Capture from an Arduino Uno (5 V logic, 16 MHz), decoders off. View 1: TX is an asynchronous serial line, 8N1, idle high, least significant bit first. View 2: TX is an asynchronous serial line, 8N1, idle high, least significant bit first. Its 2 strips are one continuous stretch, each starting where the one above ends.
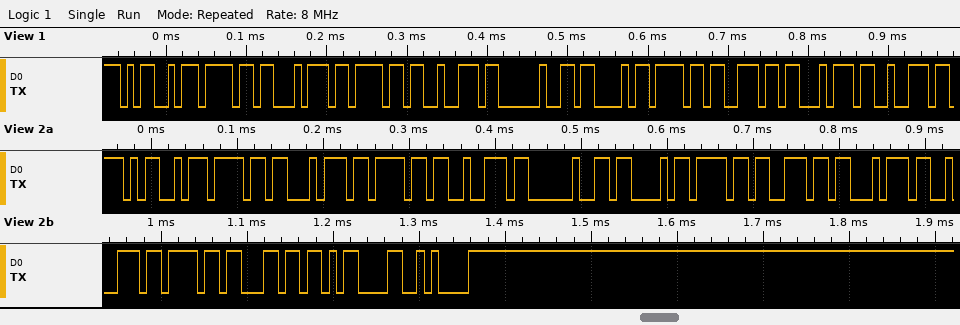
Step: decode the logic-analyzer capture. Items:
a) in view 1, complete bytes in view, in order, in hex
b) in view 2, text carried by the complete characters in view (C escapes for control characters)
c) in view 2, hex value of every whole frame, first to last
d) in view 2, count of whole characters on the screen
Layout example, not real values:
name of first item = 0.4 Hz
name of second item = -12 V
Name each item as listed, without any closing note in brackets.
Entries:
in view 1, complete bytes in view, in order, in hex = 0x4D 0x6F 0x74 0x6F 0x72 0x20 0x43 0x6F 0x6E 0x74 0x72
in view 2, text carried by the complete characters in view = "Motor Control\r\n"
in view 2, hex value of every whole frame, first to last = 4D 6F 74 6F 72 20 43 6F 6E 74 72 6F 6C 0D 0A
in view 2, count of whole characters on the screen = 15
